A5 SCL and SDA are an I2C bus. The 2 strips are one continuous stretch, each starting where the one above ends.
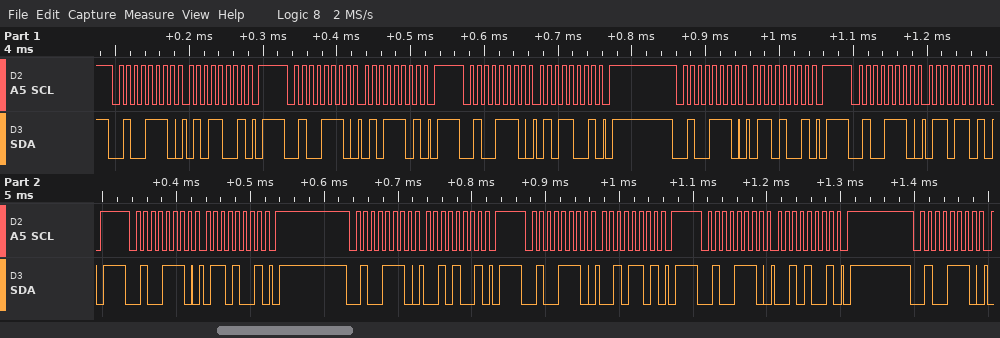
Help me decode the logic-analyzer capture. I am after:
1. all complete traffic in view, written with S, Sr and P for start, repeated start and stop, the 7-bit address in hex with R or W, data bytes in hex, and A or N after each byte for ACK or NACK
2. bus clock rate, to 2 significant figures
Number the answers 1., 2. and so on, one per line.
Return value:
1. S 27W A 59 A P S 27W A 5D A P S 27W A 59 A P S 27W A 69 A P S 27W A 6D A P S 27W A 69 A P S 27W A 29 A P S 27W A 2D A P S 27W A 29 A P S 27W A
2. 100 kHz
